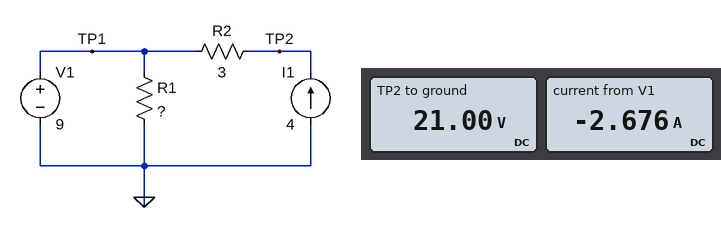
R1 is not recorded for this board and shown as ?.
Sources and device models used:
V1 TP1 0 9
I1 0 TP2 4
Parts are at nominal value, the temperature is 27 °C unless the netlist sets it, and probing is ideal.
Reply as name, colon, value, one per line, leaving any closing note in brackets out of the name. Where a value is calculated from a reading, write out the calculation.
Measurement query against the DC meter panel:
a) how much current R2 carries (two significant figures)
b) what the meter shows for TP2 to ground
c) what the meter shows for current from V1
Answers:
how much current R2 carries: (21 V - 9 V) / 3 Ω = 4.0 A
what the meter shows for TP2 to ground: 21.00 V
what the meter shows for current from V1: -2.676 A
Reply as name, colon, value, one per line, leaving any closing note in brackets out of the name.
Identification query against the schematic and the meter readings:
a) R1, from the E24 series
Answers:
R1, from the E24 series: 6.8 Ω
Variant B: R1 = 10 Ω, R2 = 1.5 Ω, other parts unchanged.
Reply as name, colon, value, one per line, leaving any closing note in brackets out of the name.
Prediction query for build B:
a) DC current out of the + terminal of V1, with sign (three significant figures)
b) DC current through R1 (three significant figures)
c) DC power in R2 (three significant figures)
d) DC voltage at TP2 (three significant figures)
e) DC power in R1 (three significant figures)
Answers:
DC current out of the + terminal of V1, with sign: -3.10 A
DC current through R1: 900 mA
DC power in R2: 24.0 W
DC voltage at TP2: 15.0 V
DC power in R1: 8.10 W
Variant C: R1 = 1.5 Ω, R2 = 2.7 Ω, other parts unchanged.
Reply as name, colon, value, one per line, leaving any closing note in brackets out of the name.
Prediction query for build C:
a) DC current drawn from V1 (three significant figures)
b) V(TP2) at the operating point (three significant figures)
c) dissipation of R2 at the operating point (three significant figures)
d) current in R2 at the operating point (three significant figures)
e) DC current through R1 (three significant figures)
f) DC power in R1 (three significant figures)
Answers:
DC current drawn from V1: 2.00 A
V(TP2) at the operating point: 19.8 V
dissipation of R2 at the operating point: 43.2 W
current in R2 at the operating point: 4.00 A
DC current through R1: 6.00 A
DC power in R1: 54.0 W
